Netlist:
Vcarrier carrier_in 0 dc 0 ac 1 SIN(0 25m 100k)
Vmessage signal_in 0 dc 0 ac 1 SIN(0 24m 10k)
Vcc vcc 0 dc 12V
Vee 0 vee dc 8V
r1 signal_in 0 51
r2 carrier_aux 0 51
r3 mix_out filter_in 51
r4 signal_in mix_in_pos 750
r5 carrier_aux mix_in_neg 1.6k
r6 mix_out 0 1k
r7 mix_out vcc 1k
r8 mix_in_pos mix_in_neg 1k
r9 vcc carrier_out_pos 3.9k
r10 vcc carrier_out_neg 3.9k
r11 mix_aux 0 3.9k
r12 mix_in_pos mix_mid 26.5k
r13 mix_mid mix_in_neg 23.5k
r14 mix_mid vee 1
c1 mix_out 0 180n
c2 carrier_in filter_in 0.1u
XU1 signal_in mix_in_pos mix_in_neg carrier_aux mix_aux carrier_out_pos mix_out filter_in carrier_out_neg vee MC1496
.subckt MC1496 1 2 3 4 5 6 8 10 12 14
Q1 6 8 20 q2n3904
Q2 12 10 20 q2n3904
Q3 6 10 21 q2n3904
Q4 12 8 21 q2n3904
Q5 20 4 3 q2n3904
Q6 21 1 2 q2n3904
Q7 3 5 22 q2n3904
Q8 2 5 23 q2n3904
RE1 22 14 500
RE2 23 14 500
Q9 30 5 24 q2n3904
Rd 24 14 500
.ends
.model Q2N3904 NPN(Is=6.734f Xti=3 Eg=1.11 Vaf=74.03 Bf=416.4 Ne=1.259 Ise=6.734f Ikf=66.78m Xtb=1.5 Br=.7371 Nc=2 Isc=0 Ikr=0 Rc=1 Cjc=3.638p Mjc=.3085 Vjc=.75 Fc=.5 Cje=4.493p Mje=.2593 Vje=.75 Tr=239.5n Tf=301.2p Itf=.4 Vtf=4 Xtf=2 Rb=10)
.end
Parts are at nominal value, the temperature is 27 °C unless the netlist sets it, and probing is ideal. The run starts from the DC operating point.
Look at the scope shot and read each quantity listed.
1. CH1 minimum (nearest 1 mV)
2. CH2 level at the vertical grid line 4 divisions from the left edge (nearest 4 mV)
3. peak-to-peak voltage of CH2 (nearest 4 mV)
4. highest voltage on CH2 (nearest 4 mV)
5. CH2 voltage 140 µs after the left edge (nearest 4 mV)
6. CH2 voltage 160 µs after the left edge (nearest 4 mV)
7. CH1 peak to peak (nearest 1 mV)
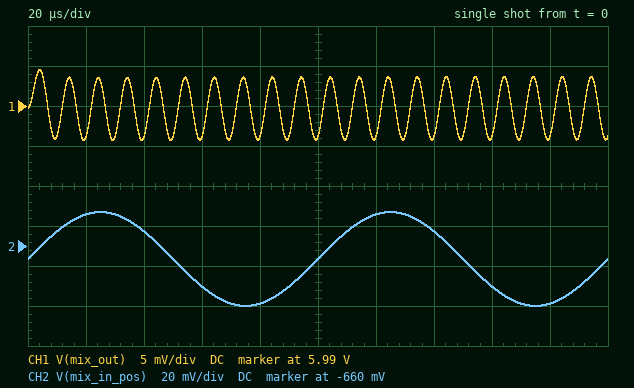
5.986 V
-688 mV
48 mV
-644 mV
-652 mV
-680 mV
9 mV
